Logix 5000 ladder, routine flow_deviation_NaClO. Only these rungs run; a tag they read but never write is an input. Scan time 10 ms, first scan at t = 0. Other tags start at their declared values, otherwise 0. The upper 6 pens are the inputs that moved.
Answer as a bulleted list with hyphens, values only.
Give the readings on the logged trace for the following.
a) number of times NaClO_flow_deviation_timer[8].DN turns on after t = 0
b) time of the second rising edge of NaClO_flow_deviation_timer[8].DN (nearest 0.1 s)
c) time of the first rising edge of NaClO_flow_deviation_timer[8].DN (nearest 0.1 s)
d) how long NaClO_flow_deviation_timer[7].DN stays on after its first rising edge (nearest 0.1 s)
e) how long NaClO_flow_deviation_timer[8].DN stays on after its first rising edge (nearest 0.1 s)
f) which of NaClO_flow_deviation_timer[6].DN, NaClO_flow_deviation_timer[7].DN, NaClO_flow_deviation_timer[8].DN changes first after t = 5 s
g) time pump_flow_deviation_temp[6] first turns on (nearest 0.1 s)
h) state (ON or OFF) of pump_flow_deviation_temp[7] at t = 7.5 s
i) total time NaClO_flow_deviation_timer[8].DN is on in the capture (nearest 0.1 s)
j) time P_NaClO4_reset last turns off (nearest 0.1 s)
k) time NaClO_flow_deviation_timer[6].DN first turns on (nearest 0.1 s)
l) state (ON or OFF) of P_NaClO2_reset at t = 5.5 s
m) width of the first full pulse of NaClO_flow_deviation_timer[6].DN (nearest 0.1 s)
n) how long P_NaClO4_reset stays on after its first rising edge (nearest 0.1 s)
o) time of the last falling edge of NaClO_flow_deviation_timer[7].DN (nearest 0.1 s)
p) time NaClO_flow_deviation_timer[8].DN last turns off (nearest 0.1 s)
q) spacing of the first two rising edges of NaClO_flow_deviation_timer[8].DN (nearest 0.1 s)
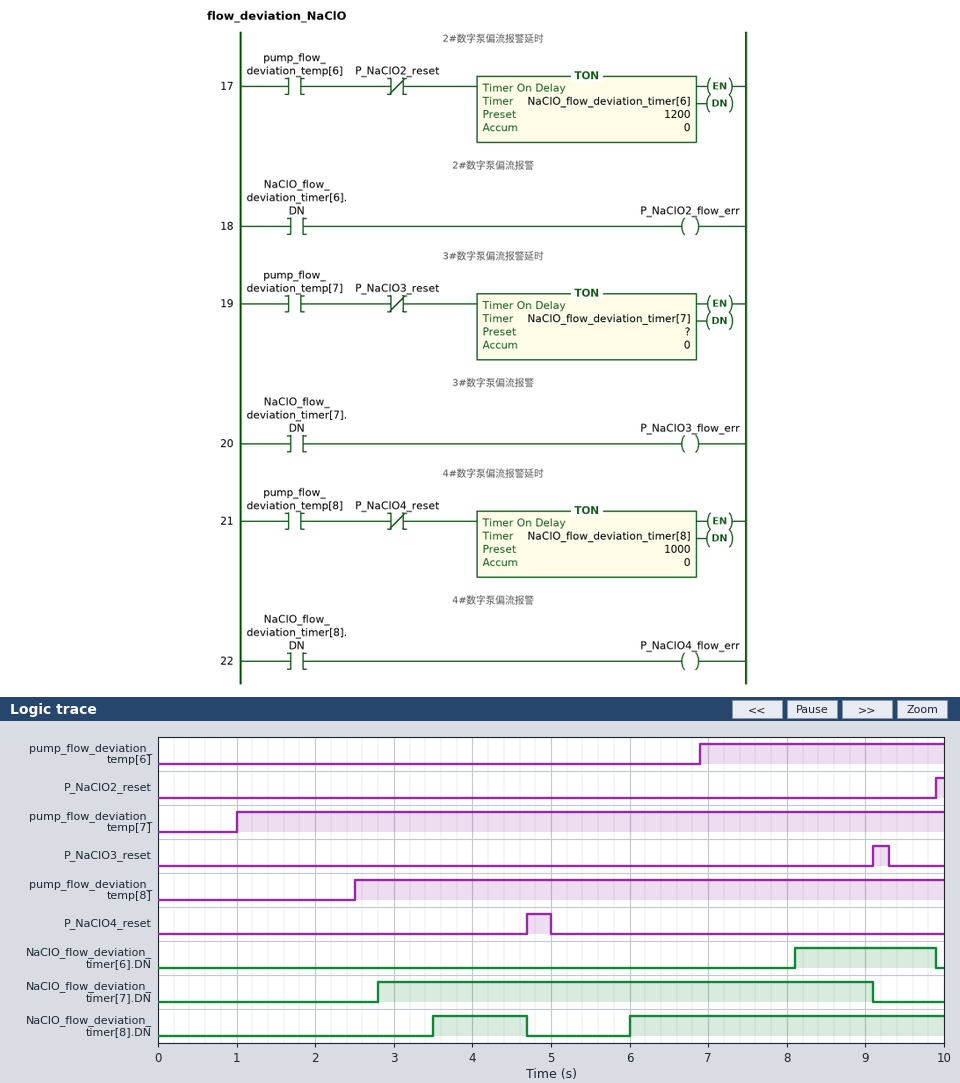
- 2
- 6.0 s
- 3.5 s
- 6.3 s
- 1.2 s
- NaClO_flow_deviation_timer[8].DN
- 6.9 s
- ON
- 5.2 s
- 5.0 s
- 8.1 s
- OFF
- 1.8 s
- 0.3 s
- 9.1 s
- 4.7 s
- 2.5 s
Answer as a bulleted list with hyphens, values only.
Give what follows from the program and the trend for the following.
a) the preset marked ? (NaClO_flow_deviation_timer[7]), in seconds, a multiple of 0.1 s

- 1.8 s
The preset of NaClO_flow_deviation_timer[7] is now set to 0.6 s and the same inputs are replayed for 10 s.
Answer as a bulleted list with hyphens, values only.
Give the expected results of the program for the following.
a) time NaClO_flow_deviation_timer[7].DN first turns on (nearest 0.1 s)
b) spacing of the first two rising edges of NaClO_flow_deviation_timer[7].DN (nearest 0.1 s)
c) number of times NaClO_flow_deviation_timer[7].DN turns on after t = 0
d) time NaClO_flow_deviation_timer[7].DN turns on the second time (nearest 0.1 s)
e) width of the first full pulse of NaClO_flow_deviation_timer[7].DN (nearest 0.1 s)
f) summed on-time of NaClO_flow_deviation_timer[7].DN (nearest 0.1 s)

- 1.6 s
- 8.3 s
- 2
- 9.9 s
- 7.5 s
- 7.6 s
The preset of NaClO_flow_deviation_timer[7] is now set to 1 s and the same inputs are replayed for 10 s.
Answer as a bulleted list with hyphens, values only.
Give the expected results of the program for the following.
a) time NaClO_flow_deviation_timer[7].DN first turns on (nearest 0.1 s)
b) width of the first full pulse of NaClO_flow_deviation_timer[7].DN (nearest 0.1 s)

- 2.0 s
- 7.1 s
